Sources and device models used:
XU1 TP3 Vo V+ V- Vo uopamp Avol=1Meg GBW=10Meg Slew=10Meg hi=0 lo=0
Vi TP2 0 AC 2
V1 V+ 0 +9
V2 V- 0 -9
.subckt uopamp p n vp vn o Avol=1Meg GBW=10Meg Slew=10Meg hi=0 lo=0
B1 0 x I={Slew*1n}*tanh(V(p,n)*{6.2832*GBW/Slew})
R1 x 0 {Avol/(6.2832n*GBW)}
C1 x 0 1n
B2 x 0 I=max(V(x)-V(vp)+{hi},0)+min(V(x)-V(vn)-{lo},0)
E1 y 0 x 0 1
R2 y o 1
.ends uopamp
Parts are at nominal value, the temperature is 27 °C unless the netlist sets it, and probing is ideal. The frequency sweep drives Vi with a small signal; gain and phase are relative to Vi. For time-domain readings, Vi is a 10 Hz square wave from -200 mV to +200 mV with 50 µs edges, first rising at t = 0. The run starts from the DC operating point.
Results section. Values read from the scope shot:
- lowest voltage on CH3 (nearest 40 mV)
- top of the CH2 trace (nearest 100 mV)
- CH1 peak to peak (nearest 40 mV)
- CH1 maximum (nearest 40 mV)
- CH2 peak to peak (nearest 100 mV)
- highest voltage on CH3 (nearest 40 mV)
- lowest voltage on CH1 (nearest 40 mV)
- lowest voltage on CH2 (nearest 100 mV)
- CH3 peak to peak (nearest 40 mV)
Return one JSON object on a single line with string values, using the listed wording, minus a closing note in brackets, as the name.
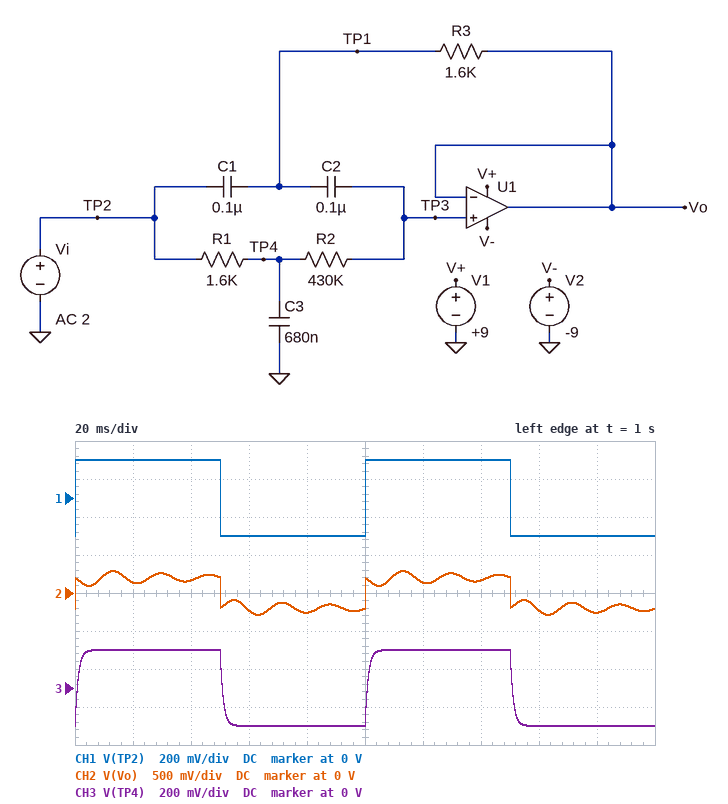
{"lowest voltage on CH3": "-200 mV", "top of the CH2 trace": "300 mV", "CH1 peak to peak": "400 mV", "CH1 maximum": "200 mV", "CH2 peak to peak": "600 mV", "highest voltage on CH3": "200 mV", "lowest voltage on CH1": "-200 mV", "lowest voltage on CH2": "-300 mV", "CH3 peak to peak": "400 mV"}
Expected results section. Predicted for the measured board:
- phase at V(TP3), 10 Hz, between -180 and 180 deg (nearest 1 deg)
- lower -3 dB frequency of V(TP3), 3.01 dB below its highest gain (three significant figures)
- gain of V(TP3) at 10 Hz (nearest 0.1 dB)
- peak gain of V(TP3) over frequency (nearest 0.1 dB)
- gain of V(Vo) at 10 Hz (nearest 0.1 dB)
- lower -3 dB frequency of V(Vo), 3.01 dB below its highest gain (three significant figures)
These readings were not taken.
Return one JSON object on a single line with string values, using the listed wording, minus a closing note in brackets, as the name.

{"phase at V(TP3), 10 Hz, between -180 and 180 deg": "-4 deg", "lower -3 dB frequency of V(TP3), 3.01 dB below its highest gain": "57.5 Hz", "gain of V(TP3) at 10 Hz": "0 dB", "peak gain of V(TP3) over frequency": "6.9 dB", "gain of V(Vo) at 10 Hz": "0 dB", "lower -3 dB frequency of V(Vo), 3.01 dB below its highest gain": "57.5 Hz"}
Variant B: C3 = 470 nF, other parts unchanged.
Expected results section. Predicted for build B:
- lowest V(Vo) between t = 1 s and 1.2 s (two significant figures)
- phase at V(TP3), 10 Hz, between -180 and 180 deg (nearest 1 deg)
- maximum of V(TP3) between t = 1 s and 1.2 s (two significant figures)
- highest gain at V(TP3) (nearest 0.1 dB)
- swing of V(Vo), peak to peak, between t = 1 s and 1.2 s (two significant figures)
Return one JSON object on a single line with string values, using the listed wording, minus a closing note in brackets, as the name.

{"lowest V(Vo) between t = 1 s and 1.2 s": "-260 mV", "phase at V(TP3), 10 Hz, between -180 and 180 deg": "-3 deg", "maximum of V(TP3) between t = 1 s and 1.2 s": "260 mV", "highest gain at V(TP3)": "2.5 dB", "swing of V(Vo), peak to peak, between t = 1 s and 1.2 s": "530 mV"}
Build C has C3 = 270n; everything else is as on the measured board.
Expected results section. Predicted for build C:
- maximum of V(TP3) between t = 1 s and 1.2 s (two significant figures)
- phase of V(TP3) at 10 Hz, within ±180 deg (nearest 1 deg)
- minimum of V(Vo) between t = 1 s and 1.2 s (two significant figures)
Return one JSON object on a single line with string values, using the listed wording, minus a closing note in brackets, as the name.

{"maximum of V(TP3) between t = 1 s and 1.2 s": "240 mV", "phase of V(TP3) at 10 Hz, within ±180 deg": "-2 deg", "minimum of V(Vo) between t = 1 s and 1.2 s": "-240 mV"}
